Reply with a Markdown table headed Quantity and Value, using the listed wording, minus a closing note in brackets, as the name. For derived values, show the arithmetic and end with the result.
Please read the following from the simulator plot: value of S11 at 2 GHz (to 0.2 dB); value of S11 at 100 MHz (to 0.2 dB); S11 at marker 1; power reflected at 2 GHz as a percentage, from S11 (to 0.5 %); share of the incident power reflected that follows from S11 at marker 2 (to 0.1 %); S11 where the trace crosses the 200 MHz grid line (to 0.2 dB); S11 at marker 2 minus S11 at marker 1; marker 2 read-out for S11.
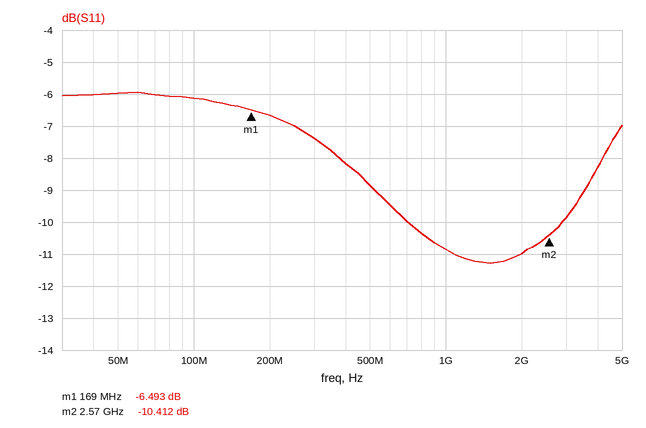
| Quantity | Value |
|---|---|
| value of S11 at 2 GHz | -11.0 dB |
| value of S11 at 100 MHz | -6.2 dB |
| S11 at marker 1 | -6.493 dB |
| power reflected at 2 GHz as a percentage, from S11 | 10^(-11/10) ≈ 7.94 %, so 8.0 % to the nearest 0.5 % |
| share of the incident power reflected that follows from S11 at marker 2 | 10^(-10.412/10) ≈ 9.1 % |
| S11 where the trace crosses the 200 MHz grid line | -6.6 dB |
| S11 at marker 2 minus S11 at marker 1 | -10.412 − (-6.493) = -3.919 dB |
| marker 2 read-out for S11 | -10.412 dB |
